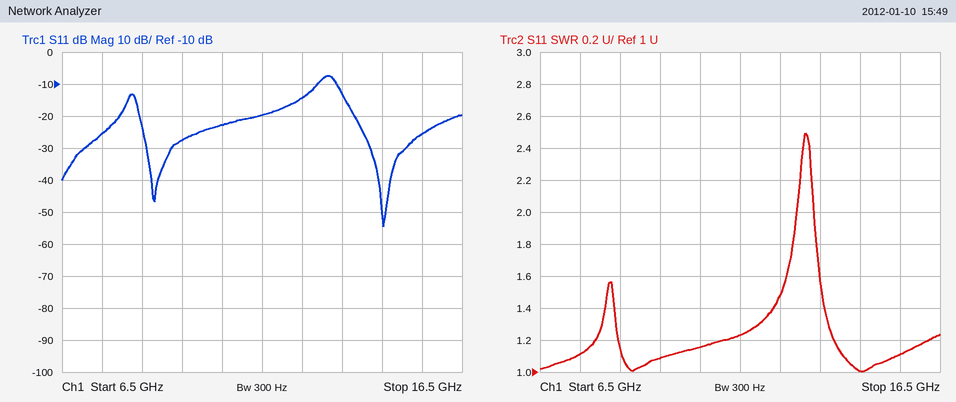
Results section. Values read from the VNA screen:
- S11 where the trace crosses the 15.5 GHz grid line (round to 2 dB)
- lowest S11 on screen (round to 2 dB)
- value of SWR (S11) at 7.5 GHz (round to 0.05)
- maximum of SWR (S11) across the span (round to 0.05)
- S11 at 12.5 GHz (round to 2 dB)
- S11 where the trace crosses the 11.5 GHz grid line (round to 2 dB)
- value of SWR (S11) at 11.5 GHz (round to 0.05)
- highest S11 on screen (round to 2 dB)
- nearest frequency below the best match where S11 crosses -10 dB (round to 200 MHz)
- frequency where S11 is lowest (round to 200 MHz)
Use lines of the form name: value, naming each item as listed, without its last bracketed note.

S11 where the trace crosses the 15.5 GHz grid line: -26 dB
lowest S11 on screen: -54 dB
value of SWR (S11) at 7.5 GHz: 1.10
maximum of SWR (S11) across the span: 2.50
S11 at 12.5 GHz: -14 dB
S11 where the trace crosses the 11.5 GHz grid line: -20 dB
value of SWR (S11) at 11.5 GHz: 1.25
highest S11 on screen: -8 dB
nearest frequency below the best match where S11 crosses -10 dB: 13.4 GHz
frequency where S11 is lowest: 14.6 GHz
